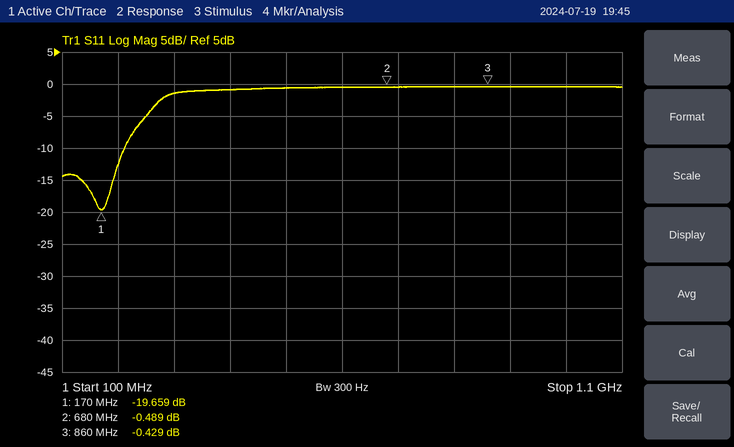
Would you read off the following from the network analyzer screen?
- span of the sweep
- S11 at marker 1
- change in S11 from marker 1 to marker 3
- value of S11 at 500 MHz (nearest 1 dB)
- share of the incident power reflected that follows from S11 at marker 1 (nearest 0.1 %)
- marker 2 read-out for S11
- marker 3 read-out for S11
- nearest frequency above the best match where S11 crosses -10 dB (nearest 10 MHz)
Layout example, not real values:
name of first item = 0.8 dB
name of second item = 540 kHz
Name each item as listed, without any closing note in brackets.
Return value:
span of the sweep = 1 GHz
S11 at marker 1 = -19.659 dB
change in S11 from marker 1 to marker 3 = 19.230 dB
value of S11 at 500 MHz = -1 dB
share of the incident power reflected that follows from S11 at marker 1 = 1.1 %
marker 2 read-out for S11 = -0.489 dB
marker 3 read-out for S11 = -0.429 dB
nearest frequency above the best match where S11 crosses -10 dB = 210 MHz
